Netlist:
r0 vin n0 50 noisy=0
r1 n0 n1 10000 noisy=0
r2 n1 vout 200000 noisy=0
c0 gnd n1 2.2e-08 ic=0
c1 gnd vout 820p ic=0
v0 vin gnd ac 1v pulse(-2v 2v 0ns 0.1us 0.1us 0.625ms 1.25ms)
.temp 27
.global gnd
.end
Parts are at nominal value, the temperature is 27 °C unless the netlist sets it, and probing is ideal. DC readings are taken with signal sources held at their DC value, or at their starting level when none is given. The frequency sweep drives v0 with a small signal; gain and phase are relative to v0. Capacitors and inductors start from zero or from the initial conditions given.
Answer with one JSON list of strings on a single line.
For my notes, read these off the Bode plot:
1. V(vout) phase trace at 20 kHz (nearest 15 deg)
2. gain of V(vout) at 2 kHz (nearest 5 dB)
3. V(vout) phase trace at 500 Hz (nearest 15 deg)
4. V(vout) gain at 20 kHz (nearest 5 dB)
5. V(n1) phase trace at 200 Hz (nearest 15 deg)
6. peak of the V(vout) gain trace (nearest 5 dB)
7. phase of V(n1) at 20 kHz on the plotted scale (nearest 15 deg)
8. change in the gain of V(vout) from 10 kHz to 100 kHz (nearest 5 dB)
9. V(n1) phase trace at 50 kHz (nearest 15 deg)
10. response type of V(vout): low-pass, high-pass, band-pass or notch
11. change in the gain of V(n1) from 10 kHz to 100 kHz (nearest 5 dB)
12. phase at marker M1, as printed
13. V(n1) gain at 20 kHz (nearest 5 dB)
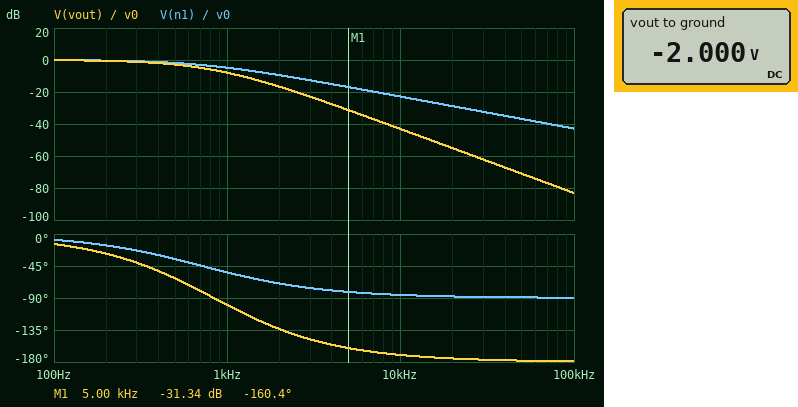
["-180 deg", "-15 dB", "-60 deg", "-55 dB", "-15 deg", "0 dB", "-90 deg", "-40 dB", "-90 deg", "low-pass", "-20 dB", "-160.4 deg", "-30 dB"]
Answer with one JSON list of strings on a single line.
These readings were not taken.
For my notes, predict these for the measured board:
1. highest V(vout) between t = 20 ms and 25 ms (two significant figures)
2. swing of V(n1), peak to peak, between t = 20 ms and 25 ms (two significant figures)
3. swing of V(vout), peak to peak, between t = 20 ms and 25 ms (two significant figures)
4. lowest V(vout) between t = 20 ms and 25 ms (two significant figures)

["1.4 V", "3.5 V", "2.8 V", "-1.4 V"]
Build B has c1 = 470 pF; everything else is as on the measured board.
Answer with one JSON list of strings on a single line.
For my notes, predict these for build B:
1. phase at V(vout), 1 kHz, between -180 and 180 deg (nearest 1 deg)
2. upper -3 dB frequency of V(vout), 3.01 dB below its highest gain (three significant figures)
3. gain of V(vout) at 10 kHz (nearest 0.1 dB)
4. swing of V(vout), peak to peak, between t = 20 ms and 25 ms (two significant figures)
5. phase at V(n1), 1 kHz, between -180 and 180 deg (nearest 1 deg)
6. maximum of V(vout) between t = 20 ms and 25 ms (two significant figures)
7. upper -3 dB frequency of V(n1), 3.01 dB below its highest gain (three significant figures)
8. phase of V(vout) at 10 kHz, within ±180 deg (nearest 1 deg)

["-85 deg", "614 Hz", "-38.4 dB", "3.2 V", "-54 deg", "1.6 V", "702 Hz", "-166 deg"]
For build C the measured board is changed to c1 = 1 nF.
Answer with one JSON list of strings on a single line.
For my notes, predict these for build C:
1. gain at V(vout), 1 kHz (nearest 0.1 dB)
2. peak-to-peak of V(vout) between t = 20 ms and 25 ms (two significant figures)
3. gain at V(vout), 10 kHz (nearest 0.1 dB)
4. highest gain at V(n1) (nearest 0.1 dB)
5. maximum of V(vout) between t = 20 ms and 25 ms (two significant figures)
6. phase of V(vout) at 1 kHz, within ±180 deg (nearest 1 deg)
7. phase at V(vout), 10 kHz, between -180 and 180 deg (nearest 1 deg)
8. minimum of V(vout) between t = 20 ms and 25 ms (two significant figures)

["-9.0 dB", "2.5 V", "-44.9 dB", "0 dB", "1.3 V", "-105 deg", "-171 deg", "-1.3 V"]
